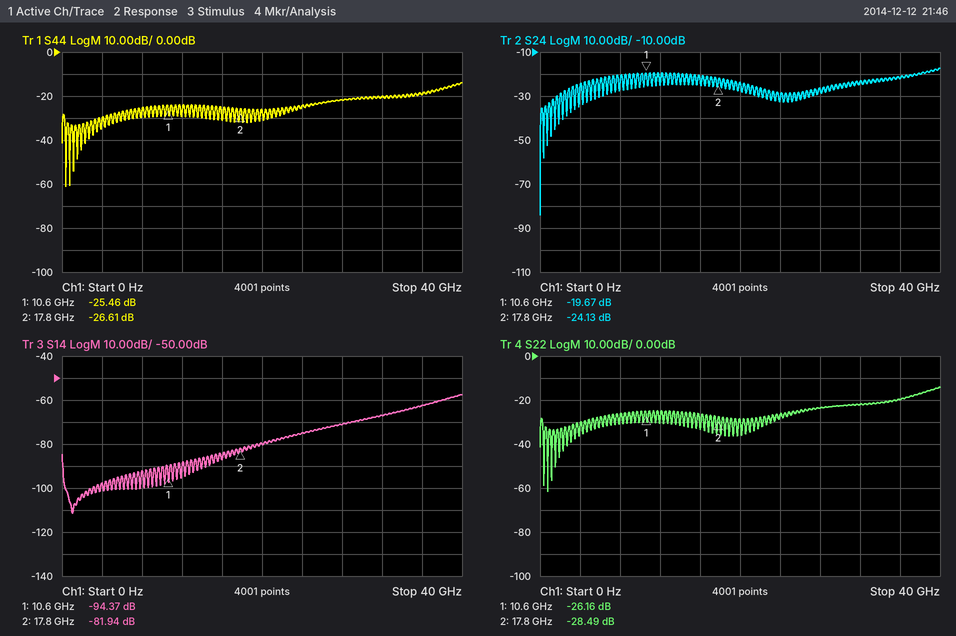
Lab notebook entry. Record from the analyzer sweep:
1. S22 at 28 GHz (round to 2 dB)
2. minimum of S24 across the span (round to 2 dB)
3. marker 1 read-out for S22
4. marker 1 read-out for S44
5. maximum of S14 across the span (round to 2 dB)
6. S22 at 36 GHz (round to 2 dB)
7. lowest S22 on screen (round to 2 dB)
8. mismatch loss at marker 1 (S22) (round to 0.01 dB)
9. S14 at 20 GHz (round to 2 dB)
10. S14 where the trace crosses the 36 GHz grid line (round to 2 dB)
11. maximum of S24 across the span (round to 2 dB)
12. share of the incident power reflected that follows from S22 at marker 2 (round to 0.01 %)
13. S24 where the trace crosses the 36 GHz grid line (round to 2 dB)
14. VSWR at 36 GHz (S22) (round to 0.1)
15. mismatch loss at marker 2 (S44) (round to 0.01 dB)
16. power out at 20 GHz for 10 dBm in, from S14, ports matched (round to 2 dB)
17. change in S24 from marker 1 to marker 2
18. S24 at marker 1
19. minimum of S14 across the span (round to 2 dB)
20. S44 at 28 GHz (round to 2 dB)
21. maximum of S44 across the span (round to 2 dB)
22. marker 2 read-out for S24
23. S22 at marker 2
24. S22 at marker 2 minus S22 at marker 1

-24 dB
-84 dB
-26.16 dB
-25.46 dB
-58 dB
-20 dB
-62 dB
0.01 dB
-80 dB
-62 dB
-18 dB
0.14 %
-22 dB
1.2
0.01 dB
-70 dBm
-4.46 dB
-19.67 dB
-112 dB
-22 dB
-14 dB
-24.13 dB
-28.49 dB
-2.33 dB
